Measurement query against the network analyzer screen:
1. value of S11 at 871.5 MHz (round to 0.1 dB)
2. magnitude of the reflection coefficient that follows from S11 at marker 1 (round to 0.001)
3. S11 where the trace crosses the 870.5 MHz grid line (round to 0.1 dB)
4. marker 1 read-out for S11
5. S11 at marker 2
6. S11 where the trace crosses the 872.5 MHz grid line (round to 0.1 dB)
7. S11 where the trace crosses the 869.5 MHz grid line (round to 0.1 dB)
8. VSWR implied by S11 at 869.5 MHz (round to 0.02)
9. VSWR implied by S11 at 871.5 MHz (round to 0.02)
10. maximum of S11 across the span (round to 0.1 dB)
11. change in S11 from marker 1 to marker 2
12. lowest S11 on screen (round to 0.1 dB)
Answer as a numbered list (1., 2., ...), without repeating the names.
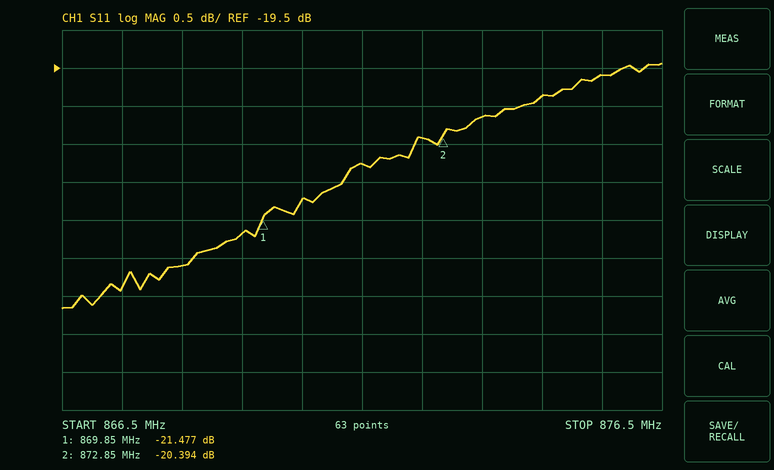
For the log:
1. -20.8 dB
2. 0.084
3. -21.2 dB
4. -21.477 dB
5. -20.394 dB
6. -20.4 dB
7. -21.7 dB
8. 1.18
9. 1.20
10. -19.4 dB
11. 1.083 dB
12. -22.7 dB
